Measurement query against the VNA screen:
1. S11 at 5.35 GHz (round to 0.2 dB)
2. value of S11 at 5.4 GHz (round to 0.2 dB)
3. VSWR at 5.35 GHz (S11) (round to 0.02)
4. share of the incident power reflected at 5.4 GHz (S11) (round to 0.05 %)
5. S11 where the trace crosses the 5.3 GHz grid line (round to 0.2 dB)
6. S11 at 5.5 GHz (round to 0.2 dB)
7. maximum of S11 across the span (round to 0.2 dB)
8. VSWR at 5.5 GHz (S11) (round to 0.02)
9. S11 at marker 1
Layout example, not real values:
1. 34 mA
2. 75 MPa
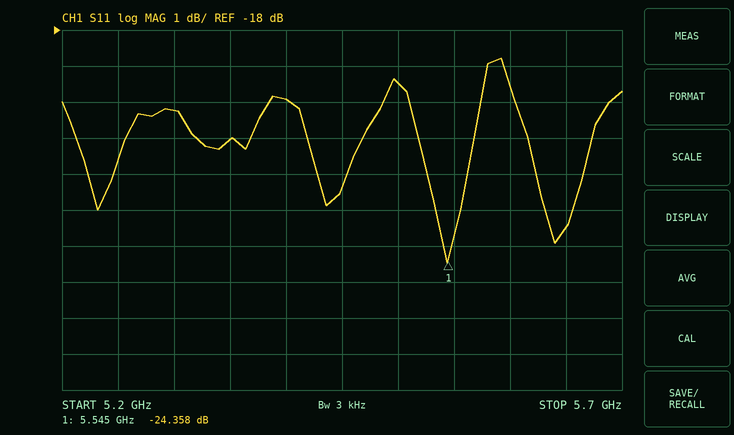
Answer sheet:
1. -21.0 dB
2. -20.0 dB
3. 1.20
4. 1.00 %
5. -20.2 dB
6. -19.4 dB
7. -18.8 dB
8. 1.24
9. -24.358 dB
